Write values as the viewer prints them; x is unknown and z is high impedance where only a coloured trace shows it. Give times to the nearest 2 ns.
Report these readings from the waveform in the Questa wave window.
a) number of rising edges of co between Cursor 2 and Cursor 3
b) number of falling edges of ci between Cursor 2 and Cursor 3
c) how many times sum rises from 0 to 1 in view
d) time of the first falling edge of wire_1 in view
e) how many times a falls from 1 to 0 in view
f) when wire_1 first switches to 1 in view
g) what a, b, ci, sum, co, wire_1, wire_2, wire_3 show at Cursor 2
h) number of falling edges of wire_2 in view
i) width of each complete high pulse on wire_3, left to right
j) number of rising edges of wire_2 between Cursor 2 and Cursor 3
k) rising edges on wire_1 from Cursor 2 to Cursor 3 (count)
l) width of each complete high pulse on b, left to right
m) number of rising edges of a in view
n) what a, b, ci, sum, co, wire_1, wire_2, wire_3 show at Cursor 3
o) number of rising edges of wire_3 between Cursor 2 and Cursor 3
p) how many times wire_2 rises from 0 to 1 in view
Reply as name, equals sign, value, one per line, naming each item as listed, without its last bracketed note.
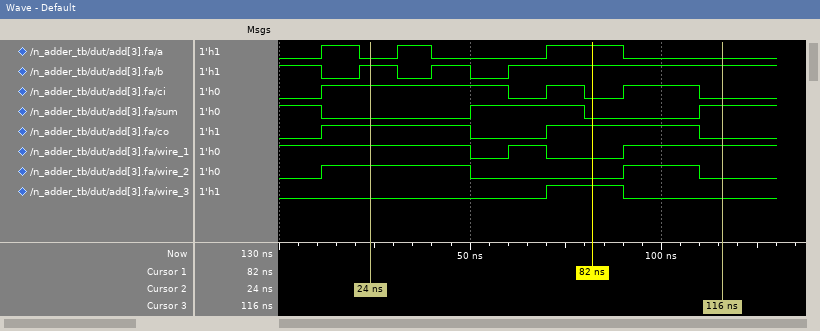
number of rising edges of co between Cursor 2 and Cursor 3 = 1
number of falling edges of ci between Cursor 2 and Cursor 3 = 3
how many times sum rises from 0 to 1 in view = 2
time of the first falling edge of wire_1 in view = 50 ns
how many times a falls from 1 to 0 in view = 3
when wire_1 first switches to 1 in view = 60 ns
what a, b, ci, sum, co, wire_1, wire_2, wire_3 show at Cursor 2 = a=0, b=1, ci=1, sum=0, co=1, wire_1=1, wire_2=1, wire_3=0
number of falling edges of wire_2 in view = 2
width of each complete high pulse on wire_3, left to right = 20 ns
number of rising edges of wire_2 between Cursor 2 and Cursor 3 = 1
rising edges on wire_1 from Cursor 2 to Cursor 3 = 2
width of each complete high pulse on b, left to right = 10 ns, 10 ns
number of rising edges of a in view = 3
what a, b, ci, sum, co, wire_1, wire_2, wire_3 show at Cursor 3 = a=0, b=1, ci=0, sum=1, co=0, wire_1=1, wire_2=0, wire_3=0
number of rising edges of wire_3 between Cursor 2 and Cursor 3 = 1
how many times wire_2 rises from 0 to 1 in view = 2
